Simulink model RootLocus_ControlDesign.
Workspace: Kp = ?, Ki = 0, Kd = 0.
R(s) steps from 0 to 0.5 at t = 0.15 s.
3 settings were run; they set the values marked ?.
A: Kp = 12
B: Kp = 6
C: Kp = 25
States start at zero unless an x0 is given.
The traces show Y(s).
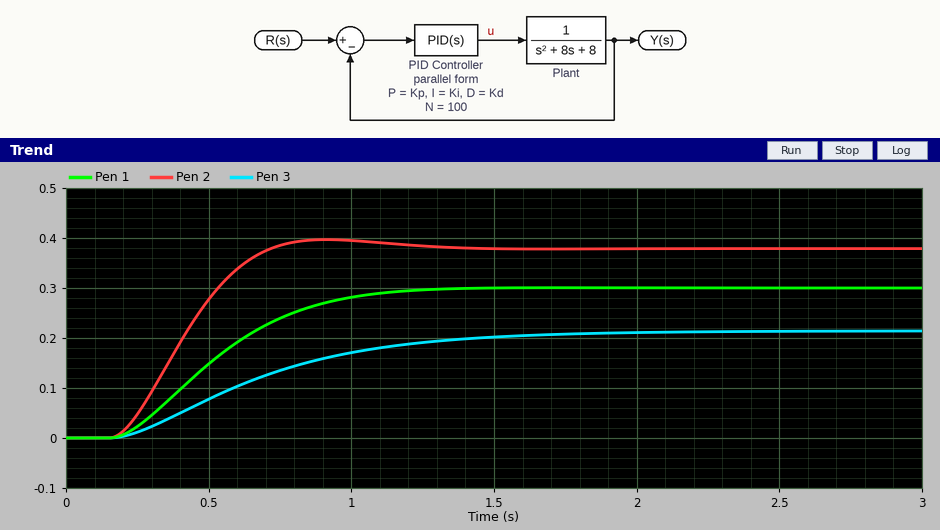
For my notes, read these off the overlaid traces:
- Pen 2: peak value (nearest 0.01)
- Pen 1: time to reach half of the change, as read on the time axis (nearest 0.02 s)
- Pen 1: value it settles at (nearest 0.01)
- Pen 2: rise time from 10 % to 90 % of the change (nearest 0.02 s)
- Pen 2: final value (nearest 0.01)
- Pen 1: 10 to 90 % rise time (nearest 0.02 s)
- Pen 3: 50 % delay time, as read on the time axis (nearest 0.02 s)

0.40
0.50 s
0.30
0.36 s
0.38
0.64 s
0.62 s
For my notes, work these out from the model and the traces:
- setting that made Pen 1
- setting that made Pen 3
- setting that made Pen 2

A
B
C
